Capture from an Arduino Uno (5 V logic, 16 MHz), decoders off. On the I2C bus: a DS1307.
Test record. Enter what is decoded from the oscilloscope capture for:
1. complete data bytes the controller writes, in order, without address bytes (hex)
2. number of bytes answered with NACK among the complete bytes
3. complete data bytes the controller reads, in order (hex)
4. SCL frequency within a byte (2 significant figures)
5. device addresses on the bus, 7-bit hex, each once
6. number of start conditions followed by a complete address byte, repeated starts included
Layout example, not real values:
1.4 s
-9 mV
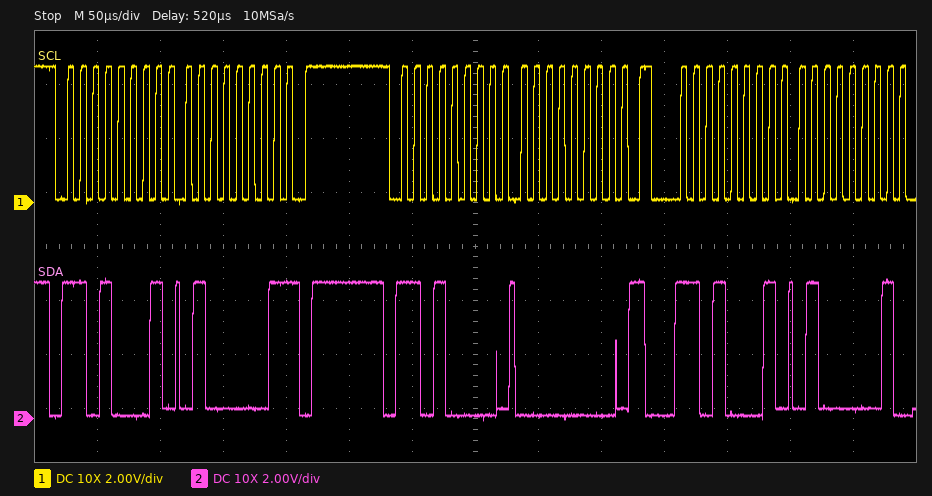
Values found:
00
1
41 41
100 kHz
0x68
3
